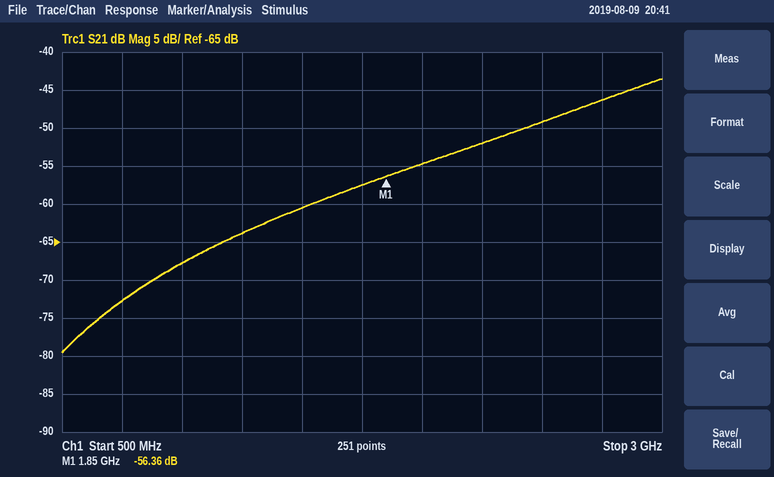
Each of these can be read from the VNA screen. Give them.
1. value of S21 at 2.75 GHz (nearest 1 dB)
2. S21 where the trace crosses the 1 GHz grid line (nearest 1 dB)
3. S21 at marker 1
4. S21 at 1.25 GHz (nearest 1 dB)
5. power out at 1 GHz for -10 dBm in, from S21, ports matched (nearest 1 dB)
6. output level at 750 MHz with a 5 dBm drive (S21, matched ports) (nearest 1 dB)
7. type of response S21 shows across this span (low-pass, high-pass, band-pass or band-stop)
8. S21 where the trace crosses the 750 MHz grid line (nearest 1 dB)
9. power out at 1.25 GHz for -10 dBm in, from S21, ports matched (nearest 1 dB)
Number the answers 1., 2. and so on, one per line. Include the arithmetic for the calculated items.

1. -46 dB
2. -68 dB
3. -56.36 dB
4. -64 dB
5. -10 dBm + (-68 dB) = -78 dBm
6. 5 dBm + (-73 dB) = -68 dBm
7. high-pass
8. -73 dB
9. -10 dBm + (-64 dB) = -74 dBm
